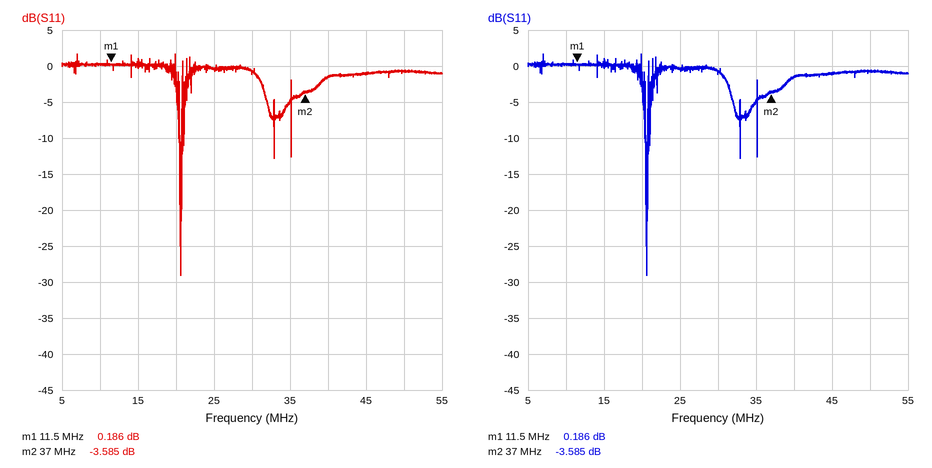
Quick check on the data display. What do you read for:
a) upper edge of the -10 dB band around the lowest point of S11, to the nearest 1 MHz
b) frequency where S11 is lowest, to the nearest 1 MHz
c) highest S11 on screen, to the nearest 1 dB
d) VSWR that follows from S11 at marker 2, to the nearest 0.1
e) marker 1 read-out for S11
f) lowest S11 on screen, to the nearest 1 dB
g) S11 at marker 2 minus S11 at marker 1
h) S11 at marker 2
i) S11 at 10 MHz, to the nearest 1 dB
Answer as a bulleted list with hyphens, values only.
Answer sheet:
- 21 MHz
- 21 MHz
- 2 dB
- 4.9
- 0.186 dB
- -29 dB
- -3.771 dB
- -3.585 dB
- 0 dB
